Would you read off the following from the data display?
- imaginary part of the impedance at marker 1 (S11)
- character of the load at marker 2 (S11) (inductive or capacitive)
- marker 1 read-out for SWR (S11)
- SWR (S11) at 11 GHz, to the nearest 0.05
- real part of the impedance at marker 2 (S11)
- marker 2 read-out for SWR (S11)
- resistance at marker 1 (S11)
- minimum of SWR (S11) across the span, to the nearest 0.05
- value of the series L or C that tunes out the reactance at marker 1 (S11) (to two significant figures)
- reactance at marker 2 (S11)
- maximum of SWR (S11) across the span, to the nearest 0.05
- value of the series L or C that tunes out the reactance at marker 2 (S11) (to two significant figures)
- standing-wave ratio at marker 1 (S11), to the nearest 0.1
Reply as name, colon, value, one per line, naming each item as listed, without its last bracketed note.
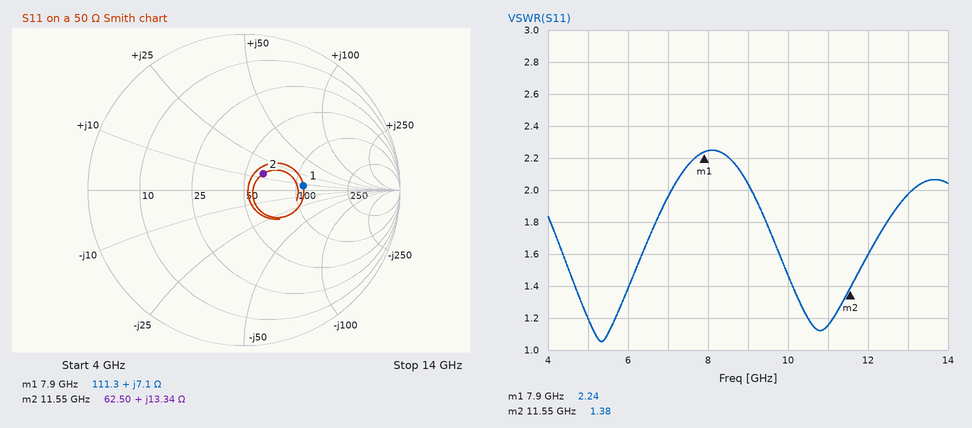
imaginary part of the impedance at marker 1: +7.1 Ω
character of the load at marker 2 (S11): inductive
marker 1 read-out for SWR: 2.24
SWR (S11) at 11 GHz, to the nearest 0.05: 1.15
real part of the impedance at marker 2: 62.50 Ω
marker 2 read-out for SWR: 1.38
resistance at marker 1: 111.3 Ω
minimum of SWR (S11) across the span, to the nearest 0.05: 1.05
value of the series L or C that tunes out the reactance at marker 1 (S11): 2.8 pF
reactance at marker 2: +13.34 Ω
maximum of SWR (S11) across the span, to the nearest 0.05: 2.25
value of the series L or C that tunes out the reactance at marker 2 (S11): 1.0 pF
standing-wave ratio at marker 1 (S11), to the nearest 0.1: 2.2
